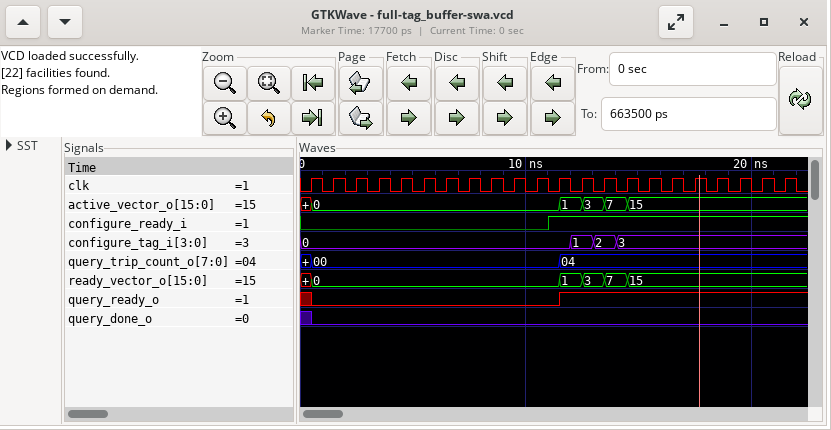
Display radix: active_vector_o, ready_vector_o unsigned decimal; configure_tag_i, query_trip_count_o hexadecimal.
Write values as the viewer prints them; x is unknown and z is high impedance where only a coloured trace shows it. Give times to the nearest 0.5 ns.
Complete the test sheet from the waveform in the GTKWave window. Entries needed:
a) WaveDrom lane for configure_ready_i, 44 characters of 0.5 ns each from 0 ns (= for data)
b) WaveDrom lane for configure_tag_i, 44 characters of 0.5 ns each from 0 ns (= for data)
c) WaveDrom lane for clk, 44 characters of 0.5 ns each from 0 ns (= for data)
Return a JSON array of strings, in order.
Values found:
["{name: 'configure_ready_i', wave: '0.....................1.....................'}", "{name: 'configure_tag_i', wave: '=.......................=.=.=...............', data: '0 1 2 3'}", "{name: 'clk', wave: '01010101010101010101010101010101010101010101'}"]
